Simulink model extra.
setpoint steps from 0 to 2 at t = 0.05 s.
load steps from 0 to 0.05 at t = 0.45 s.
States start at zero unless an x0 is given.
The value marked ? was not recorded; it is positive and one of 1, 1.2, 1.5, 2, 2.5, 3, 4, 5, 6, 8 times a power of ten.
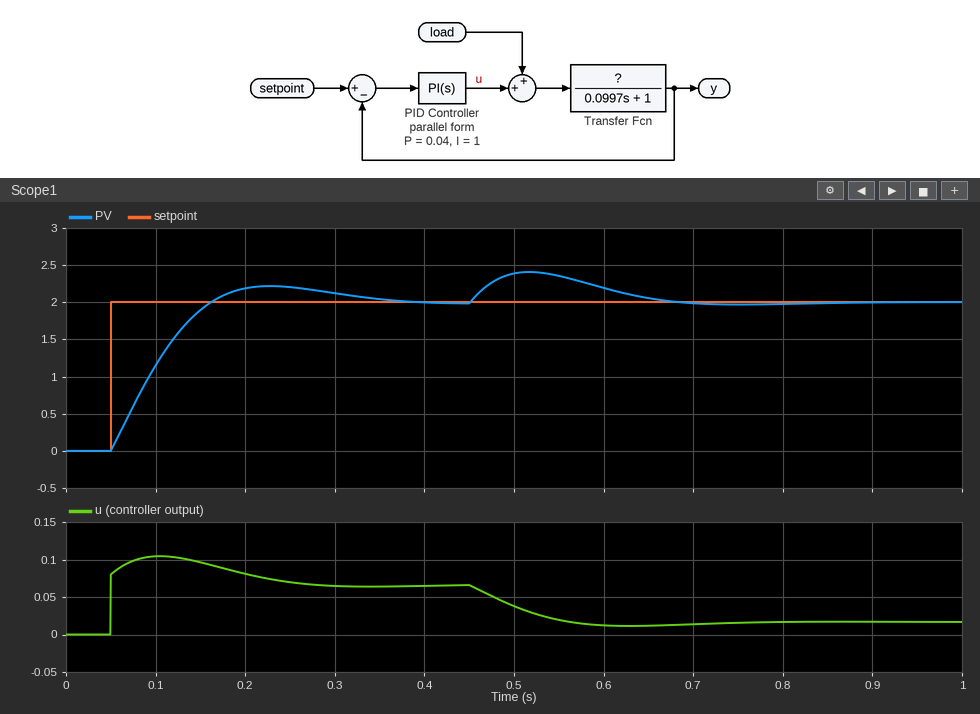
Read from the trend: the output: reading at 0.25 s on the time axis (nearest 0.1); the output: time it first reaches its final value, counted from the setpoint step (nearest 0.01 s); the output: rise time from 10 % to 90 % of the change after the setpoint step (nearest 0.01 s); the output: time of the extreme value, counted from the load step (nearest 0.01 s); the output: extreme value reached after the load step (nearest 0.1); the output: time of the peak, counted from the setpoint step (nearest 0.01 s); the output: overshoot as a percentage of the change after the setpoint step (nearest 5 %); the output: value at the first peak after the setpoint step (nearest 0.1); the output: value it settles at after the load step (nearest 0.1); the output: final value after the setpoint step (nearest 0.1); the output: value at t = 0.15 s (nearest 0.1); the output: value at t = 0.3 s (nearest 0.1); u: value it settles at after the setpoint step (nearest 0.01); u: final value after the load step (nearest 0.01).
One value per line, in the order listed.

2.2
0.11 s
0.08 s
0.07 s
2.4
0.18 s
10 %
2.2
2.0
2.0
1.9
2.1
0.07
0.02
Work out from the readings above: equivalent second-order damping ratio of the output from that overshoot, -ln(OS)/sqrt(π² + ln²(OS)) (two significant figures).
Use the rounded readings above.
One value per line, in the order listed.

0.59
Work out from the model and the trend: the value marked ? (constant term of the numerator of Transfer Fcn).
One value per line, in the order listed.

30
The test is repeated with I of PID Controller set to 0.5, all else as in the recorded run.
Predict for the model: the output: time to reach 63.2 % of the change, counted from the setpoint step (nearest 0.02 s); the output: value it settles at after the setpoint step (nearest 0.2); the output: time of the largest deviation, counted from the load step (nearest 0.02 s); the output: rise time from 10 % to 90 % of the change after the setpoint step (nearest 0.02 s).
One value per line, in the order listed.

0.08 s
2.0
0.08 s
0.14 s
